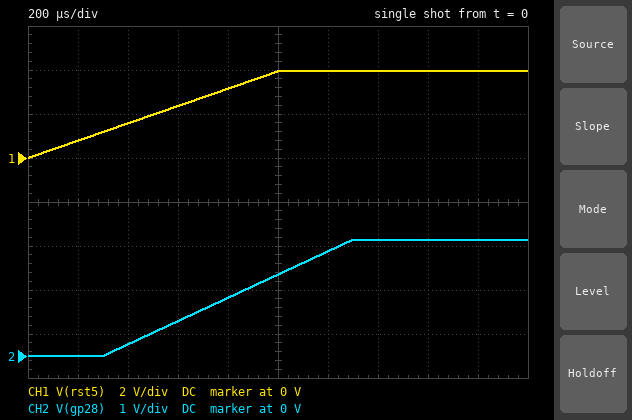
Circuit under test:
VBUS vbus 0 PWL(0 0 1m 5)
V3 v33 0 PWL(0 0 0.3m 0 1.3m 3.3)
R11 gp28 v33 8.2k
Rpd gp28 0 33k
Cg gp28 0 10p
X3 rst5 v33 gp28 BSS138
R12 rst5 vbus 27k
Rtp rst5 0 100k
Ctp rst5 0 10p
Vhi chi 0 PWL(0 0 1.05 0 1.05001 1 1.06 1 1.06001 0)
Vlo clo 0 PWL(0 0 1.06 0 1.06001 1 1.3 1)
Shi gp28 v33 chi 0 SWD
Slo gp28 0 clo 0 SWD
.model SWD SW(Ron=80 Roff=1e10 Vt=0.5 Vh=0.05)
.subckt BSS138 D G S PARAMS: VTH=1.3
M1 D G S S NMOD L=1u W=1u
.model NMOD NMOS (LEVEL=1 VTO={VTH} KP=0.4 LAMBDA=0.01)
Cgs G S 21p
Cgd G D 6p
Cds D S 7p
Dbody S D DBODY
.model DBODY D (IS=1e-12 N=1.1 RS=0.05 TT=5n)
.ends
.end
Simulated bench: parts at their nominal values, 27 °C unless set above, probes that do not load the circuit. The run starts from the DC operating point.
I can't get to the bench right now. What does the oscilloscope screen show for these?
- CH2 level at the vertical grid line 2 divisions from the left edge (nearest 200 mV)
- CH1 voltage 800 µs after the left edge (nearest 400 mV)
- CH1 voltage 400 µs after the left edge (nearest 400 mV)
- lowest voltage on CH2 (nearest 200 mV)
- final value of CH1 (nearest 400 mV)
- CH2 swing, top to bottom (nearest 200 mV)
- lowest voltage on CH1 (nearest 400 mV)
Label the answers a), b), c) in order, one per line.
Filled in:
a) 200 mV
b) 3.2 V
c) 1.6 V
d) 0 V
e) 4.0 V
f) 2.6 V
g) 0 V
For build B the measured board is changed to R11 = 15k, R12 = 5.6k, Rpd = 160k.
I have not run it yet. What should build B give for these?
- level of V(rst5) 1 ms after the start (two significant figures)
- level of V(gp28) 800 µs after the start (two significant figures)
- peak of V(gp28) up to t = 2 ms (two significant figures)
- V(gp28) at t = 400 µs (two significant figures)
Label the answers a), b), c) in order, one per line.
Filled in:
a) 4.7 V
b) 1.5 V
c) 3.0 V
d) 300 mV
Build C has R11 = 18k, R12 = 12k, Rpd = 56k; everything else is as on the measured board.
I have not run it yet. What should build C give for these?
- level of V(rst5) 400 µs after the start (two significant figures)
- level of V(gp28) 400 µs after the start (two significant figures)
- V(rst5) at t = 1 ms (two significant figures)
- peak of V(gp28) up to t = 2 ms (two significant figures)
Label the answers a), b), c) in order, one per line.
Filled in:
a) 1.8 V
b) 250 mV
c) 4.5 V
d) 2.5 V
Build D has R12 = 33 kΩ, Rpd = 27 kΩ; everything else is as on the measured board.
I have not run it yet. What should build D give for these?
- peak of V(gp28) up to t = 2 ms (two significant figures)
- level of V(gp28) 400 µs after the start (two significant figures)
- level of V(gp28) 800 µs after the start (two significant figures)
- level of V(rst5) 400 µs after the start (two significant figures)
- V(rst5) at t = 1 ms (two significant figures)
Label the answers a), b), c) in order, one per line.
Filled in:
a) 2.5 V
b) 250 mV
c) 1.3 V
d) 1.5 V
e) 3.8 V
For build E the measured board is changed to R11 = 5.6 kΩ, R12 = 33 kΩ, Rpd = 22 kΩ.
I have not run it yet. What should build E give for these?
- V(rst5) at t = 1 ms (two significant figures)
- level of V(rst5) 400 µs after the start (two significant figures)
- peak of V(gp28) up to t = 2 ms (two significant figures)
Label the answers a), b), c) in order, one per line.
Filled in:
a) 3.8 V
b) 1.5 V
c) 2.6 V
